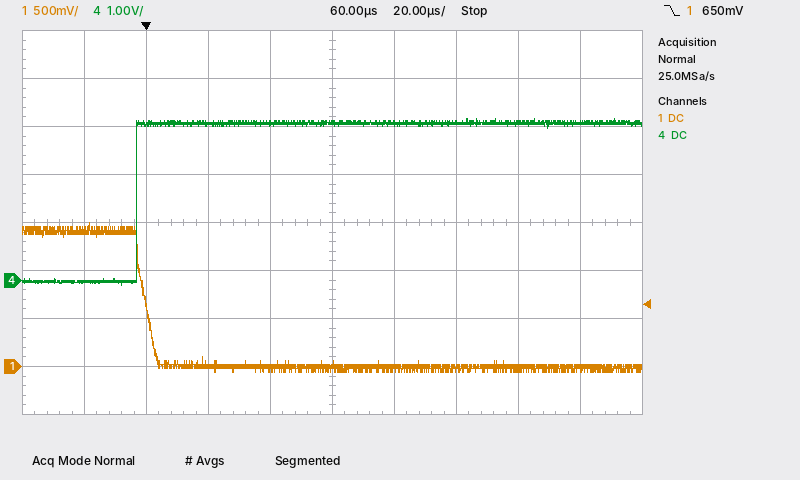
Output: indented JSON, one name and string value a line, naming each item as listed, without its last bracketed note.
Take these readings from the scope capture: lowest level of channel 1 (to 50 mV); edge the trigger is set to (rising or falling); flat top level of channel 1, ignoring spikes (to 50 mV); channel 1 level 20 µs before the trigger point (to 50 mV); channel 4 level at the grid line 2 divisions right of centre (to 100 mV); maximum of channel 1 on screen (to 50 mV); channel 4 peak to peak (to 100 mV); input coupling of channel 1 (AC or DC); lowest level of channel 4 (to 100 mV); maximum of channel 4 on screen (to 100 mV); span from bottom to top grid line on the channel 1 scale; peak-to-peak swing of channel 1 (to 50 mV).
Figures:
{
  "lowest level of channel 1": "-50 mV",
  "edge the trigger is set to": "falling",
  "flat top level of channel 1, ignoring spikes": "1.40 V",
  "channel 1 level 20 µs before the trigger point": "1.40 V",
  "channel 4 level at the grid line 2 divisions right of centre": "3.3 V",
  "maximum of channel 1 on screen": "1.50 V",
  "channel 4 peak to peak": "3.5 V",
  "input coupling of channel 1": "DC",
  "lowest level of channel 4": "-100 mV",
  "maximum of channel 4 on screen": "3.4 V",
  "span from bottom to top grid line on the channel 1 scale": "4 V",
  "peak-to-peak swing of channel 1": "1.55 V"
}
